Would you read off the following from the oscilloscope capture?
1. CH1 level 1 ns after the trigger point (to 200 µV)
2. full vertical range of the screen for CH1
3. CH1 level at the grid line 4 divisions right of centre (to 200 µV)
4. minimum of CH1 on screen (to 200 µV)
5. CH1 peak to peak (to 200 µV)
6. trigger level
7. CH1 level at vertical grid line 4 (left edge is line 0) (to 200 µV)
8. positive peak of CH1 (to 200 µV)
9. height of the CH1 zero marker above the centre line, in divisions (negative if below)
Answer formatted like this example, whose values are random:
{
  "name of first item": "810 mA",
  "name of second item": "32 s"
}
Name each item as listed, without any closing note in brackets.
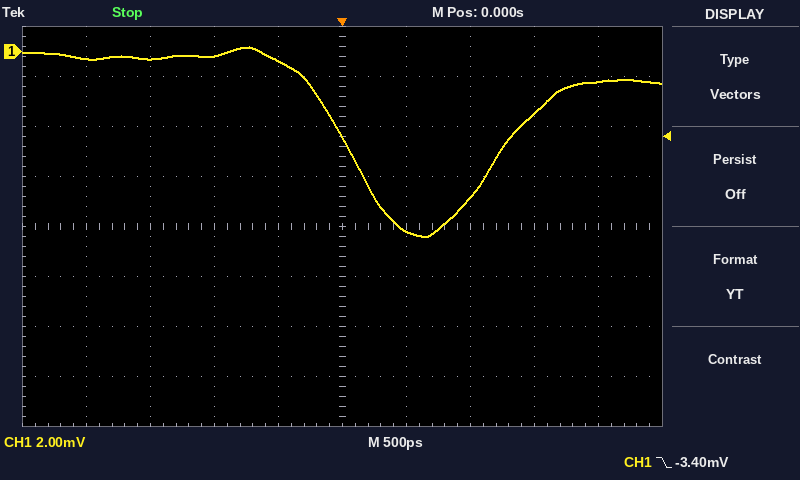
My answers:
{
  "CH1 level 1 ns after the trigger point": "-5.8 mV",
  "full vertical range of the screen for CH1": "16 mV",
  "CH1 level at the grid line 4 divisions right of centre": "-1.2 mV",
  "minimum of CH1 on screen": "-7.4 mV",
  "CH1 peak to peak": "7.6 mV",
  "trigger level": "-3.40 mV",
  "CH1 level at vertical grid line 4 (left edge is line 0)": "-400 µV",
  "positive peak of CH1": "200 µV",
  "height of the CH1 zero marker above the centre line, in divisions": "+3.5 div"
}
